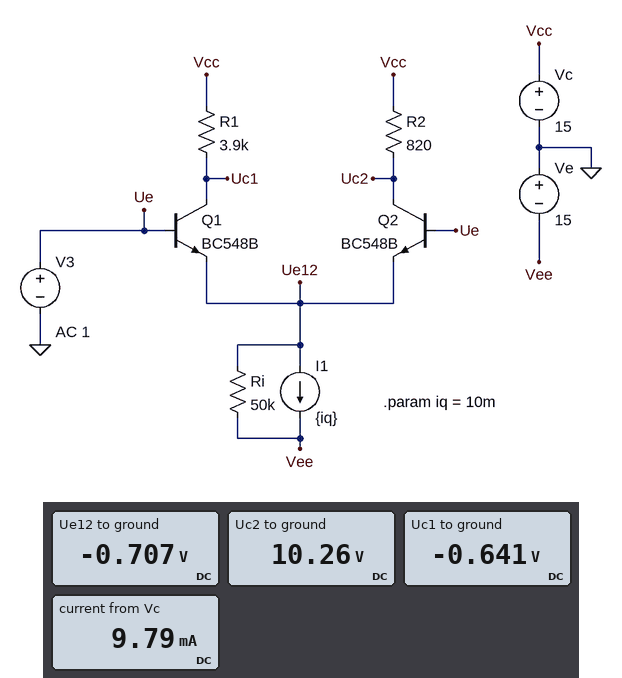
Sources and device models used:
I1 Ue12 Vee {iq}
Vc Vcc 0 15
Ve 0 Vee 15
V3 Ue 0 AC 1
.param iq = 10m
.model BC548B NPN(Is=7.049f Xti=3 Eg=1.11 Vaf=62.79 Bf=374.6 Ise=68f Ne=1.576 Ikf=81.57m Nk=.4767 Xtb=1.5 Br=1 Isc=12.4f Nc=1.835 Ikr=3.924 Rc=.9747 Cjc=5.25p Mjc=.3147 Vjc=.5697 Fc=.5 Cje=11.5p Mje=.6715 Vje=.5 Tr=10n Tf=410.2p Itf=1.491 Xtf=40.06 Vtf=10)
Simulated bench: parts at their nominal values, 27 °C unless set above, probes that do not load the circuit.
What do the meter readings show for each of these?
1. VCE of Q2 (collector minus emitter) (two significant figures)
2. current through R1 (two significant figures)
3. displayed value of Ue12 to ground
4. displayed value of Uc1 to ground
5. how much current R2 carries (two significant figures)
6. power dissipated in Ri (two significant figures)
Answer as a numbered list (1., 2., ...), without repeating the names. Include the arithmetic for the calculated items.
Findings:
1. 10.26 V - (-707 mV) = 11 V
2. (15 V - (-641 mV)) / 3.9 kΩ = 4.0 mA
3. -0.707 V
4. -0.641 V
5. (15 V - 10.26 V) / 820 Ω = 5.8 mA
6. (-707 mV - (-15 V))^2 / 50 kΩ = 4.1 mW
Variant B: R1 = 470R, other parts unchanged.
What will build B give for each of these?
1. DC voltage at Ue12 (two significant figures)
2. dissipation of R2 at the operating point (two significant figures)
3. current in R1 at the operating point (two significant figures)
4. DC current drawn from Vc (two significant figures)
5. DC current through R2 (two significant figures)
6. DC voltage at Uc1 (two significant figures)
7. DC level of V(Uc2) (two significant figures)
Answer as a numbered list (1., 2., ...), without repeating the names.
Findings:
1. -700 mV
2. 21 mW
3. 5.2 mA
4. 10 mA
5. 5.1 mA
6. 13 V
7. 11 V
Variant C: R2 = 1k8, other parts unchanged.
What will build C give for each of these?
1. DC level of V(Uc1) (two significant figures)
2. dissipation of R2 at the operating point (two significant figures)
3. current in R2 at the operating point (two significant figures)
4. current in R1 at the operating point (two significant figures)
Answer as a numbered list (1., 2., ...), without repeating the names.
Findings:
1. -650 mV
2. 57 mW
3. 5.6 mA
4. 4.0 mA
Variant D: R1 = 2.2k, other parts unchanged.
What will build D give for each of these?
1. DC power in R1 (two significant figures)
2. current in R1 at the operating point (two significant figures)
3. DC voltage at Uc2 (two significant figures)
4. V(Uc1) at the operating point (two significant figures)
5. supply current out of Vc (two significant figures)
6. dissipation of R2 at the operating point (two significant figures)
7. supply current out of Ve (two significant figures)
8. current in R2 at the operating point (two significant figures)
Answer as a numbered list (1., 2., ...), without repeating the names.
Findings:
1. 53 mW
2. 4.9 mA
3. 11 V
4. 4.2 V
5. 10 mA
6. 24 mW
7. 10 mA
8. 5.4 mA
